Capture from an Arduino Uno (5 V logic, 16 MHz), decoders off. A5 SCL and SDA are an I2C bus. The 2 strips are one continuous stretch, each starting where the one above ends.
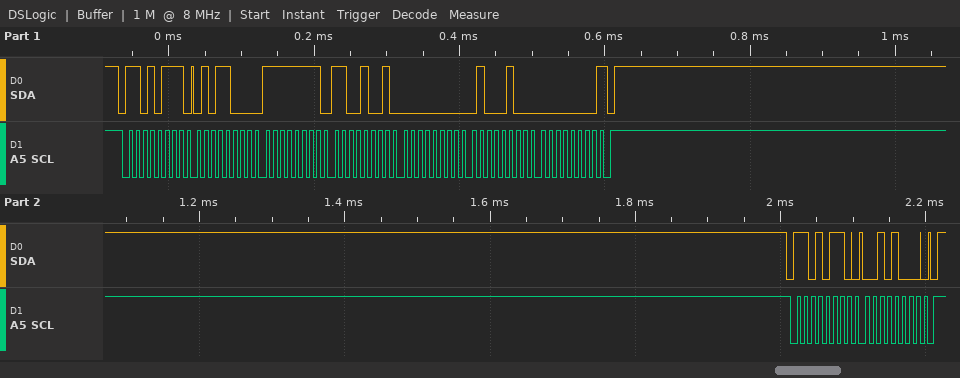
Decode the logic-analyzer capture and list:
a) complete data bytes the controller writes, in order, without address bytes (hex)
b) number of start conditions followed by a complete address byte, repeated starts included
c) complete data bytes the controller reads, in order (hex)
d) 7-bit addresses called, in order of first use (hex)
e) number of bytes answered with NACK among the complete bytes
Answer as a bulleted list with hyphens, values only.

- 28
- 2
- 58 FF C9 00 44 00
- 0x6B
- 1
